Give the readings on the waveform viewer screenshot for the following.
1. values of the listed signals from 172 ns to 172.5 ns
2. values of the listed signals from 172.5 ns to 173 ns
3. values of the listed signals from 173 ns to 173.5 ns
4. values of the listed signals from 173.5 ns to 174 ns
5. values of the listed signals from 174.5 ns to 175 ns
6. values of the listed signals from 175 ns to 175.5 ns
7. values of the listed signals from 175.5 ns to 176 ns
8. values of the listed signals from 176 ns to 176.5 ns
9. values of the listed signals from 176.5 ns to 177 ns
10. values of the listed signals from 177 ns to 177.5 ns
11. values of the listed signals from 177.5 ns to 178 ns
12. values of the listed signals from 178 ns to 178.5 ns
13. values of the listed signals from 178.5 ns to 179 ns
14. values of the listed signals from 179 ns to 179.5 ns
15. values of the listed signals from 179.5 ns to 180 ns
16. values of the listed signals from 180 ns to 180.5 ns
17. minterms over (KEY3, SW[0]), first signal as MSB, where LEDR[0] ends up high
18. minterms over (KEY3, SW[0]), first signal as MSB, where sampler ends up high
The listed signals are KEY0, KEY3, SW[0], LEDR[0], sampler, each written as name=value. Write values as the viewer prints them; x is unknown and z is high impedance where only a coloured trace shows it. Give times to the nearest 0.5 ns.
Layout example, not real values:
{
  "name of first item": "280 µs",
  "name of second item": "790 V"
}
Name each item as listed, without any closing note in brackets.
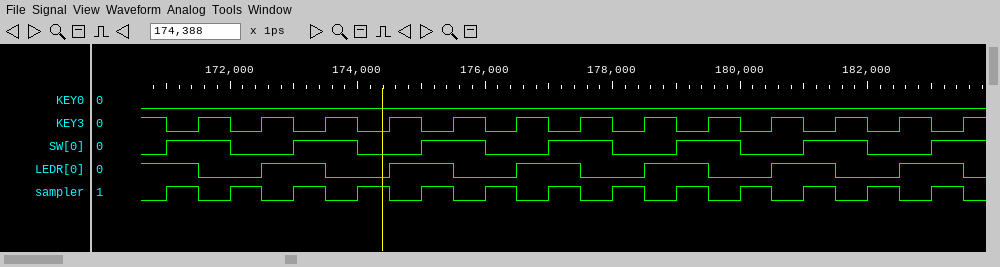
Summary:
{
  "values of the listed signals from 172 ns to 172.5 ns": "KEY0=0, KEY3=0, SW[0]=0, LEDR[0]=0, sampler=1",
  "values of the listed signals from 172.5 ns to 173 ns": "KEY0=0, KEY3=1, SW[0]=0, LEDR[0]=1, sampler=0",
  "values of the listed signals from 173 ns to 173.5 ns": "KEY0=0, KEY3=0, SW[0]=1, LEDR[0]=1, sampler=1",
  "values of the listed signals from 173.5 ns to 174 ns": "KEY0=0, KEY3=1, SW[0]=1, LEDR[0]=0, sampler=0",
  "values of the listed signals from 174.5 ns to 175 ns": "KEY0=0, KEY3=1, SW[0]=0, LEDR[0]=1, sampler=0",
  "values of the listed signals from 175 ns to 175.5 ns": "KEY0=0, KEY3=0, SW[0]=1, LEDR[0]=1, sampler=1",
  "values of the listed signals from 175.5 ns to 176 ns": "KEY0=0, KEY3=1, SW[0]=1, LEDR[0]=0, sampler=0",
  "values of the listed signals from 176 ns to 176.5 ns": "KEY0=0, KEY3=0, SW[0]=0, LEDR[0]=0, sampler=1",
  "values of the listed signals from 176.5 ns to 177 ns": "KEY0=0, KEY3=1, SW[0]=0, LEDR[0]=1, sampler=0",
  "values of the listed signals from 177 ns to 177.5 ns": "KEY0=0, KEY3=0, SW[0]=1, LEDR[0]=1, sampler=1",
  "values of the listed signals from 177.5 ns to 178 ns": "KEY0=0, KEY3=1, SW[0]=1, LEDR[0]=0, sampler=0",
  "values of the listed signals from 178 ns to 178.5 ns": "KEY0=0, KEY3=0, SW[0]=0, LEDR[0]=0, sampler=1",
  "values of the listed signals from 178.5 ns to 179 ns": "KEY0=0, KEY3=1, SW[0]=0, LEDR[0]=1, sampler=0",
  "values of the listed signals from 179 ns to 179.5 ns": "KEY0=0, KEY3=0, SW[0]=1, LEDR[0]=1, sampler=1",
  "values of the listed signals from 179.5 ns to 180 ns": "KEY0=0, KEY3=1, SW[0]=1, LEDR[0]=0, sampler=0",
  "values of the listed signals from 180 ns to 180.5 ns": "KEY0=0, KEY3=0, SW[0]=0, LEDR[0]=0, sampler=1",
  "minterms over (KEY3, SW[0]), first signal as MSB, where LEDR[0] ends up high": "1, 2",
  "minterms over (KEY3, SW[0]), first signal as MSB, where sampler ends up high": "0, 1"
}
